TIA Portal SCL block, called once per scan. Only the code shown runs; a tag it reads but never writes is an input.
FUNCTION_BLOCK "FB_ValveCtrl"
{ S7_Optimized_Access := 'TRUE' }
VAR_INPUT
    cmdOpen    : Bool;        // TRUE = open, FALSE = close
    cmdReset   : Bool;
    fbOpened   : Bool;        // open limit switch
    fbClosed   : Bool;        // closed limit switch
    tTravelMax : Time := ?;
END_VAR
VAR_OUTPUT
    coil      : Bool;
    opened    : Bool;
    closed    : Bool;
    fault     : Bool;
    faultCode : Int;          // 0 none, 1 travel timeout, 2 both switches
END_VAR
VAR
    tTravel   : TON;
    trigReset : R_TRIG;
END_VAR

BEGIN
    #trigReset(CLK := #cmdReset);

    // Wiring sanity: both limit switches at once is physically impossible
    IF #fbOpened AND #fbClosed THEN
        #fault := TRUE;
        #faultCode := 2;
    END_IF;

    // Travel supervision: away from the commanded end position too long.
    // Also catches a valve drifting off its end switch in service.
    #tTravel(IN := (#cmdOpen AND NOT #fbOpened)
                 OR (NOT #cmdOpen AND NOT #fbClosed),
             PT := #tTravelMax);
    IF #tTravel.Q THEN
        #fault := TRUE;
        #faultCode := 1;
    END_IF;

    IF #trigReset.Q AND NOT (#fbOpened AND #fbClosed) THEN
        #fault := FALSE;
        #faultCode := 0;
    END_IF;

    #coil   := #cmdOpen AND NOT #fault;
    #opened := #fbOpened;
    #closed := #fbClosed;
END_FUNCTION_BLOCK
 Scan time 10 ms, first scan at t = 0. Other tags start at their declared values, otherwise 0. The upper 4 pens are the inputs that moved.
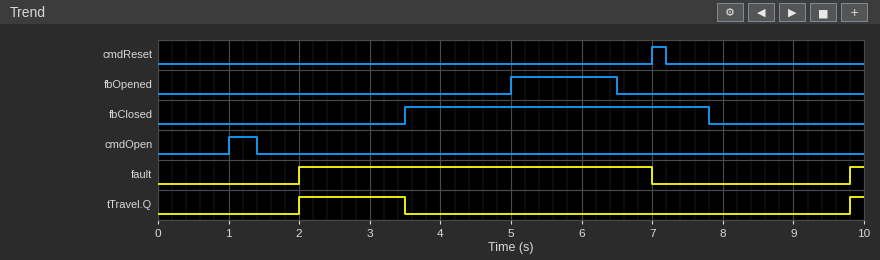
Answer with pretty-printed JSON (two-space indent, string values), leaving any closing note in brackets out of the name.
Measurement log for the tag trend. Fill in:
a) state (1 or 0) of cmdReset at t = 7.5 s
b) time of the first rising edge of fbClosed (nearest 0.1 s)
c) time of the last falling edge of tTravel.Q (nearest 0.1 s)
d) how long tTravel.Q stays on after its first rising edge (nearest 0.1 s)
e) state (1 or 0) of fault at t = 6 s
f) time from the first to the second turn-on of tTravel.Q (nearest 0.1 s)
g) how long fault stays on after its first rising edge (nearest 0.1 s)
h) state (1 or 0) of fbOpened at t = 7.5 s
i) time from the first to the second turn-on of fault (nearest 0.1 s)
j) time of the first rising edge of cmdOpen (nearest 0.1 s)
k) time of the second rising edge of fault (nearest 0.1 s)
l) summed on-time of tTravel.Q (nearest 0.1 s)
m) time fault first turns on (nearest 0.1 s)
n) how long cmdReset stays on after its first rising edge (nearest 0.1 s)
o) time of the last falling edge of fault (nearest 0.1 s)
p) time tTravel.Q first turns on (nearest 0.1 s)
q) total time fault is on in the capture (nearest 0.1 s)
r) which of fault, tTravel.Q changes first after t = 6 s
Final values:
{
  "state (1 or 0) of cmdReset at t = 7.5 s": "0",
  "time of the first rising edge of fbClosed": "3.5 s",
  "time of the last falling edge of tTravel.Q": "3.5 s",
  "how long tTravel.Q stays on after its first rising edge": "1.5 s",
  "state (1 or 0) of fault at t = 6 s": "1",
  "time from the first to the second turn-on of tTravel.Q": "7.8 s",
  "how long fault stays on after its first rising edge": "5.0 s",
  "state (1 or 0) of fbOpened at t = 7.5 s": "0",
  "time from the first to the second turn-on of fault": "7.8 s",
  "time of the first rising edge of cmdOpen": "1.0 s",
  "time of the second rising edge of fault": "9.8 s",
  "summed on-time of tTravel.Q": "1.7 s",
  "time fault first turns on": "2.0 s",
  "how long cmdReset stays on after its first rising edge": "0.2 s",
  "time of the last falling edge of fault": "7.0 s",
  "time tTravel.Q first turns on": "2.0 s",
  "total time fault is on in the capture": "5.2 s",
  "which of fault, tTravel.Q changes first after t = 6 s": "fault"
}
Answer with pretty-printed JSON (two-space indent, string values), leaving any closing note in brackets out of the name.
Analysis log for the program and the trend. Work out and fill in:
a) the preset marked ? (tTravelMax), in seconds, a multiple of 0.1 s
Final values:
{
  "the preset marked ? (tTravelMax), in seconds, a multiple of 0.1 s": "2.0 s"
}
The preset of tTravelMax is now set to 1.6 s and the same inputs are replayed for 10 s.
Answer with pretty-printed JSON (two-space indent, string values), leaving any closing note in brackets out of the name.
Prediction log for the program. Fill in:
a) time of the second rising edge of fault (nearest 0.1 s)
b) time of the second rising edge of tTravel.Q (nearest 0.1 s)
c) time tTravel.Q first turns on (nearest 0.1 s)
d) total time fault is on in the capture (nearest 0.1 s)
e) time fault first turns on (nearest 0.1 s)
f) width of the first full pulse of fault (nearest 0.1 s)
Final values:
{
  "time of the second rising edge of fault": "9.4 s",
  "time of the second rising edge of tTravel.Q": "9.4 s",
  "time tTravel.Q first turns on": "1.6 s",
  "total time fault is on in the capture": "6.0 s",
  "time fault first turns on": "1.6 s",
  "width of the first full pulse of fault": "5.4 s"
}
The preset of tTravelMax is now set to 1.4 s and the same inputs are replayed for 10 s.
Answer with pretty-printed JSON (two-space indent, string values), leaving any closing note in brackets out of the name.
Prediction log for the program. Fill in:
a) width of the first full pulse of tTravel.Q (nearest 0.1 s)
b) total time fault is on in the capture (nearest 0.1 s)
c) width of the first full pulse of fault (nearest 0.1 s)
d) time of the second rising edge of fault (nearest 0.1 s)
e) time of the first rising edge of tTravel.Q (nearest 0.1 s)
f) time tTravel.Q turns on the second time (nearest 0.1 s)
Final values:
{
  "width of the first full pulse of tTravel.Q": "2.1 s",
  "total time fault is on in the capture": "6.4 s",
  "width of the first full pulse of fault": "5.6 s",
  "time of the second rising edge of fault": "9.2 s",
  "time of the first rising edge of tTravel.Q": "1.4 s",
  "time tTravel.Q turns on the second time": "9.2 s"
}
